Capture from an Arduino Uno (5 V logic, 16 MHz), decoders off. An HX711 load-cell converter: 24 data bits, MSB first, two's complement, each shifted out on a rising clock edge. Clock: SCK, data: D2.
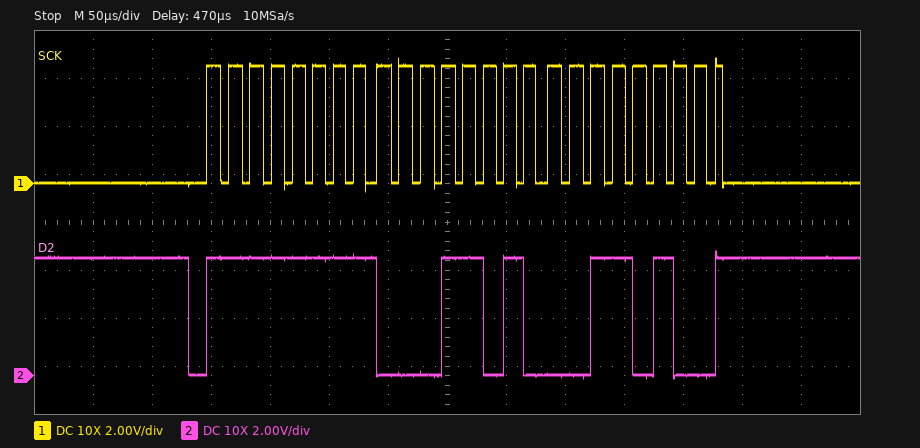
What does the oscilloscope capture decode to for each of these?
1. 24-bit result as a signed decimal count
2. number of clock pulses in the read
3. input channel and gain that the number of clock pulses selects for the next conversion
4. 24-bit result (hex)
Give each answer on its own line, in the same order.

-58828
25
channel A, gain 128
0xFF1A34
